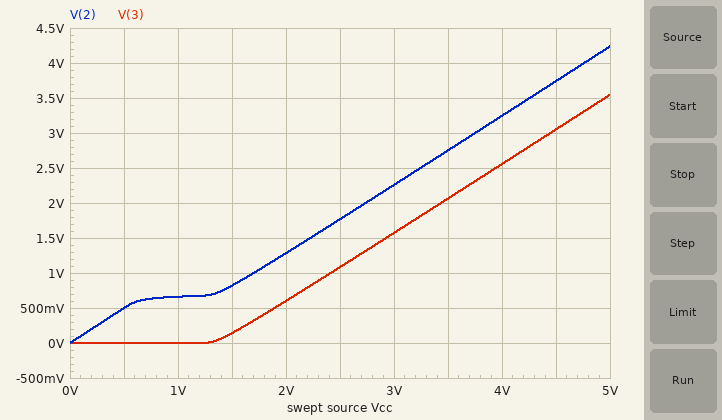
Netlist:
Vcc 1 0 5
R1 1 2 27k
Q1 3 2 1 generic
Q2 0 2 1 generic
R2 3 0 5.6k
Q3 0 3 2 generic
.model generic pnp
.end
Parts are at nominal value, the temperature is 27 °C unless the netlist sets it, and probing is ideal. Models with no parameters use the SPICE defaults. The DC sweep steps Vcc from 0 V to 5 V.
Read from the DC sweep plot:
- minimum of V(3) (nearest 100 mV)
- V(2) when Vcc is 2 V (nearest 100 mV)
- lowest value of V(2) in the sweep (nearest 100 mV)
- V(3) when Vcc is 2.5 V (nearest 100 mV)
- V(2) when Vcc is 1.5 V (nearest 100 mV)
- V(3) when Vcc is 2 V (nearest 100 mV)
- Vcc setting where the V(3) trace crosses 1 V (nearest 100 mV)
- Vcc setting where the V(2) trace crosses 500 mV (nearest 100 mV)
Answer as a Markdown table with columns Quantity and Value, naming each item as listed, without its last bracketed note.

| Quantity | Value |
|---|---|
| minimum of V(3) | 0 V |
| V(2) when Vcc is 2 V | 1.3 V |
| lowest value of V(2) in the sweep | 0 V |
| V(3) when Vcc is 2.5 V | 1.1 V |
| V(2) when Vcc is 1.5 V | 800 mV |
| V(3) when Vcc is 2 V | 600 mV |
| Vcc setting where the V(3) trace crosses 1 V | 2.4 V |
| Vcc setting where the V(2) trace crosses 500 mV | 500 mV |
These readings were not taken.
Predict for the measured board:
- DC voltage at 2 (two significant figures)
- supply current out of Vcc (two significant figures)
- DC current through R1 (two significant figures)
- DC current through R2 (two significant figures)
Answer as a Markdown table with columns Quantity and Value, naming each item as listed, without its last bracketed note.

| Quantity | Value |
|---|---|
| DC voltage at 2 | 4.2 V |
| supply current out of Vcc | 1.3 mA |
| DC current through R1 | 28 µA |
| DC current through R2 | 630 µA |
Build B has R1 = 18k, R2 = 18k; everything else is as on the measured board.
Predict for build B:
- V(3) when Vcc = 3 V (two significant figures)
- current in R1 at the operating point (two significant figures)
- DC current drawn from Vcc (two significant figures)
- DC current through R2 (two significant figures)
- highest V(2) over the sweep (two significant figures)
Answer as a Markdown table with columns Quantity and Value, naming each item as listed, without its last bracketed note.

| Quantity | Value |
|---|---|
| V(3) when Vcc = 3 V | 1.6 V |
| current in R1 at the operating point | 41 µA |
| DC current drawn from Vcc | 440 µA |
| DC current through R2 | 200 µA |
| highest V(2) over the sweep | 4.3 V |
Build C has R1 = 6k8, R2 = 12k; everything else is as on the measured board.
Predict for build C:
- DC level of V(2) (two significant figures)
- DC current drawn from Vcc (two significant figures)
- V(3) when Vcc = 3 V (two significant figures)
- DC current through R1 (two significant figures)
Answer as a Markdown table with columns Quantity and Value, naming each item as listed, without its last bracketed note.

| Quantity | Value |
|---|---|
| DC level of V(2) | 4.3 V |
| DC current drawn from Vcc | 700 µA |
| V(3) when Vcc = 3 V | 1.6 V |
| DC current through R1 | 110 µA |
